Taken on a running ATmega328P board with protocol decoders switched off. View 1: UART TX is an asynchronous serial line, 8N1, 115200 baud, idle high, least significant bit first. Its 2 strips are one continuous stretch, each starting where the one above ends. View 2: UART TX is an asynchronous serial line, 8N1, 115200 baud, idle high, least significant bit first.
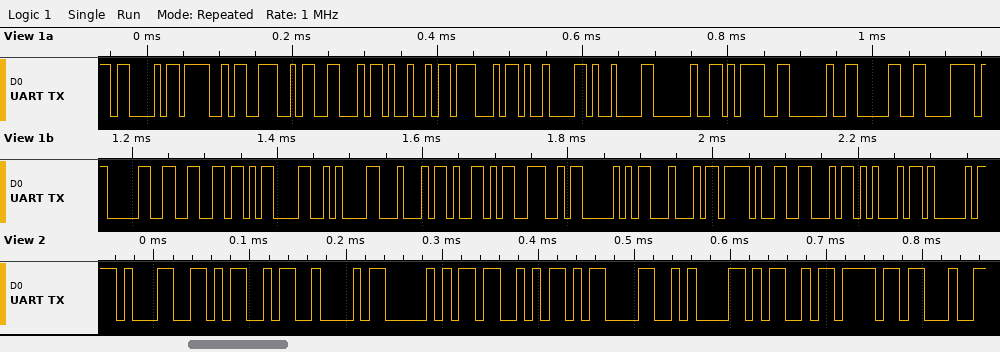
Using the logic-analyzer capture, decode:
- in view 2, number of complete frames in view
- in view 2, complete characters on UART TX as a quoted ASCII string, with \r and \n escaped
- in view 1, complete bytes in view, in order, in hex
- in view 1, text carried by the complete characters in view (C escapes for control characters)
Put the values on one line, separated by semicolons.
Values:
9; "1MBPS\r\nMo"; 43 4F 4E 46 49 47 09 09 20 3D 20 30 78 30 66 0D 0A 44 59 4E 50 44 2F 46 45 41; "CONFIG\t\t = 0x0f\r\nDYNPD/FEA"
